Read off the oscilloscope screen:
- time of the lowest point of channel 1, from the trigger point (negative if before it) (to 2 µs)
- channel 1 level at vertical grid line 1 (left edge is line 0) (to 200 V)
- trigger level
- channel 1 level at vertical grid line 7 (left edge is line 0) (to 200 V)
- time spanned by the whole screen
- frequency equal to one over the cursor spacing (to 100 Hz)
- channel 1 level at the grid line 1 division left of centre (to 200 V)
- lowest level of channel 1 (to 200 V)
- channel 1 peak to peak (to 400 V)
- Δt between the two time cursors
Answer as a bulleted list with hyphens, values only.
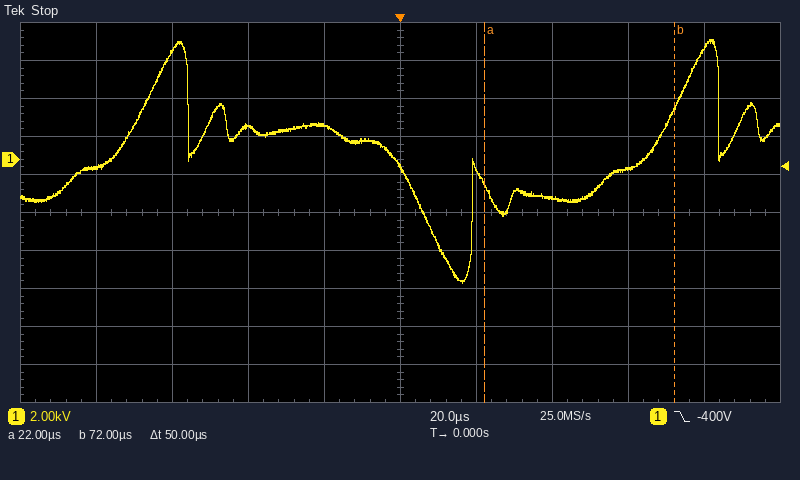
- +16 µs
- -400 V
- -400 V
- -2.0 kV
- 200 µs
- 20.0 kHz
- 1.8 kV
- -6.6 kV
- 12.8 kV
- 50 µs
